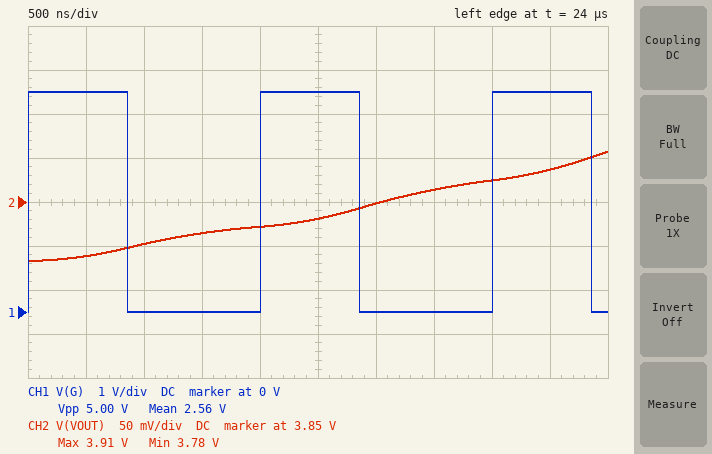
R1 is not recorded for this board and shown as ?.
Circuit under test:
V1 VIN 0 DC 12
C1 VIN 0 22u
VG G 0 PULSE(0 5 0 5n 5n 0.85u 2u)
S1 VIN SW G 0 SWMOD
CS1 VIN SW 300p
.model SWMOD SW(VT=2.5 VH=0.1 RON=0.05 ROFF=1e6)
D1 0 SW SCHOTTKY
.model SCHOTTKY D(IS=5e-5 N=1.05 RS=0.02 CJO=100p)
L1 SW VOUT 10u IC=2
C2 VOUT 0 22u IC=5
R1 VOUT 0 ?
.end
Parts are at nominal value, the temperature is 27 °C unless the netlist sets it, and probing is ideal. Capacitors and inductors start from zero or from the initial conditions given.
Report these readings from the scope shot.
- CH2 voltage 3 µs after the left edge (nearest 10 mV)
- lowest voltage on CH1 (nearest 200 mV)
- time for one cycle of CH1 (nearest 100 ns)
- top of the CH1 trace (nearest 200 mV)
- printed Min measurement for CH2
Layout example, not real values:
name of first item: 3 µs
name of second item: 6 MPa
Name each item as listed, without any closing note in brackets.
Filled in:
CH2 voltage 3 µs after the left edge: 3.85 V
lowest voltage on CH1: 0 V
time for one cycle of CH1: 2.0 µs
top of the CH1 trace: 5.0 V
printed Min measurement for CH2: 3.78 V
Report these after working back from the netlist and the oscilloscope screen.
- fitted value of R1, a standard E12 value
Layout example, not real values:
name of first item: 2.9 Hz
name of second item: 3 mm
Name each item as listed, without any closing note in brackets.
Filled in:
fitted value of R1, a standard E12 value: 1 Ω
